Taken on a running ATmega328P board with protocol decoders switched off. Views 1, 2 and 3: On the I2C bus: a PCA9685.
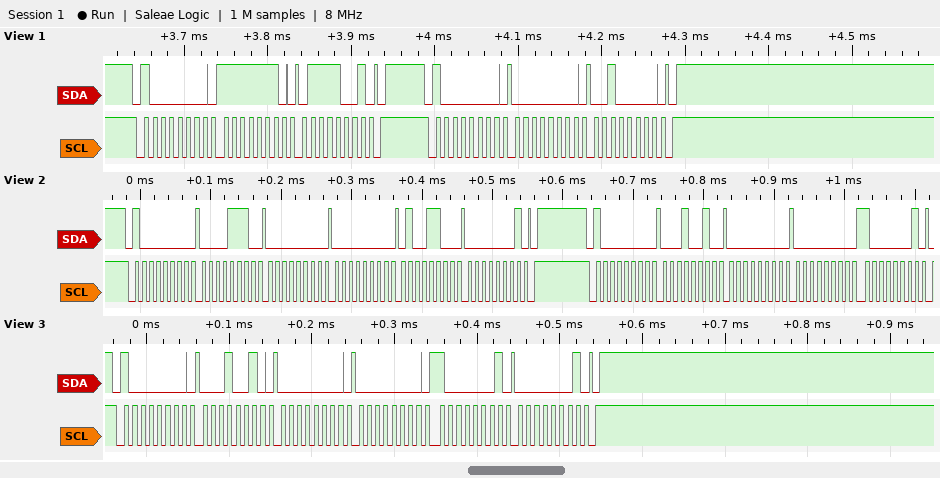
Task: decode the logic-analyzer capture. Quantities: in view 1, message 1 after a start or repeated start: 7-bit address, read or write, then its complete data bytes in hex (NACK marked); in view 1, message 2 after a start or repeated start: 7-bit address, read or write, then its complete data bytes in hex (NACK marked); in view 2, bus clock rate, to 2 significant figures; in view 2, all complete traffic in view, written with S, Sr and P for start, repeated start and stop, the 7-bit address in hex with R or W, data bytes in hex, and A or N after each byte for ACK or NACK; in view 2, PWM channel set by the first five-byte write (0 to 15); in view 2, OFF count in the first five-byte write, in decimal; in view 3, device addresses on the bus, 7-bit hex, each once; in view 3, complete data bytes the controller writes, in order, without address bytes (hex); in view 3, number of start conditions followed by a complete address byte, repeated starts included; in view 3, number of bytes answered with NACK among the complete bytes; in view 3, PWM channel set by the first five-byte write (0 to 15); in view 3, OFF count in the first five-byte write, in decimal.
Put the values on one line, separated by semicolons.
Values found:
0x40 write: FE 79; 0x40 write: 00 20; 100 kHz; S 40W A 0E A 00 A 00 A 4C A 01 A P S 40W A 12 A 00 A 00 A 81 A; 2; 332; 0x40; 12 00 00 81 01; 1; 0; 3; 385
